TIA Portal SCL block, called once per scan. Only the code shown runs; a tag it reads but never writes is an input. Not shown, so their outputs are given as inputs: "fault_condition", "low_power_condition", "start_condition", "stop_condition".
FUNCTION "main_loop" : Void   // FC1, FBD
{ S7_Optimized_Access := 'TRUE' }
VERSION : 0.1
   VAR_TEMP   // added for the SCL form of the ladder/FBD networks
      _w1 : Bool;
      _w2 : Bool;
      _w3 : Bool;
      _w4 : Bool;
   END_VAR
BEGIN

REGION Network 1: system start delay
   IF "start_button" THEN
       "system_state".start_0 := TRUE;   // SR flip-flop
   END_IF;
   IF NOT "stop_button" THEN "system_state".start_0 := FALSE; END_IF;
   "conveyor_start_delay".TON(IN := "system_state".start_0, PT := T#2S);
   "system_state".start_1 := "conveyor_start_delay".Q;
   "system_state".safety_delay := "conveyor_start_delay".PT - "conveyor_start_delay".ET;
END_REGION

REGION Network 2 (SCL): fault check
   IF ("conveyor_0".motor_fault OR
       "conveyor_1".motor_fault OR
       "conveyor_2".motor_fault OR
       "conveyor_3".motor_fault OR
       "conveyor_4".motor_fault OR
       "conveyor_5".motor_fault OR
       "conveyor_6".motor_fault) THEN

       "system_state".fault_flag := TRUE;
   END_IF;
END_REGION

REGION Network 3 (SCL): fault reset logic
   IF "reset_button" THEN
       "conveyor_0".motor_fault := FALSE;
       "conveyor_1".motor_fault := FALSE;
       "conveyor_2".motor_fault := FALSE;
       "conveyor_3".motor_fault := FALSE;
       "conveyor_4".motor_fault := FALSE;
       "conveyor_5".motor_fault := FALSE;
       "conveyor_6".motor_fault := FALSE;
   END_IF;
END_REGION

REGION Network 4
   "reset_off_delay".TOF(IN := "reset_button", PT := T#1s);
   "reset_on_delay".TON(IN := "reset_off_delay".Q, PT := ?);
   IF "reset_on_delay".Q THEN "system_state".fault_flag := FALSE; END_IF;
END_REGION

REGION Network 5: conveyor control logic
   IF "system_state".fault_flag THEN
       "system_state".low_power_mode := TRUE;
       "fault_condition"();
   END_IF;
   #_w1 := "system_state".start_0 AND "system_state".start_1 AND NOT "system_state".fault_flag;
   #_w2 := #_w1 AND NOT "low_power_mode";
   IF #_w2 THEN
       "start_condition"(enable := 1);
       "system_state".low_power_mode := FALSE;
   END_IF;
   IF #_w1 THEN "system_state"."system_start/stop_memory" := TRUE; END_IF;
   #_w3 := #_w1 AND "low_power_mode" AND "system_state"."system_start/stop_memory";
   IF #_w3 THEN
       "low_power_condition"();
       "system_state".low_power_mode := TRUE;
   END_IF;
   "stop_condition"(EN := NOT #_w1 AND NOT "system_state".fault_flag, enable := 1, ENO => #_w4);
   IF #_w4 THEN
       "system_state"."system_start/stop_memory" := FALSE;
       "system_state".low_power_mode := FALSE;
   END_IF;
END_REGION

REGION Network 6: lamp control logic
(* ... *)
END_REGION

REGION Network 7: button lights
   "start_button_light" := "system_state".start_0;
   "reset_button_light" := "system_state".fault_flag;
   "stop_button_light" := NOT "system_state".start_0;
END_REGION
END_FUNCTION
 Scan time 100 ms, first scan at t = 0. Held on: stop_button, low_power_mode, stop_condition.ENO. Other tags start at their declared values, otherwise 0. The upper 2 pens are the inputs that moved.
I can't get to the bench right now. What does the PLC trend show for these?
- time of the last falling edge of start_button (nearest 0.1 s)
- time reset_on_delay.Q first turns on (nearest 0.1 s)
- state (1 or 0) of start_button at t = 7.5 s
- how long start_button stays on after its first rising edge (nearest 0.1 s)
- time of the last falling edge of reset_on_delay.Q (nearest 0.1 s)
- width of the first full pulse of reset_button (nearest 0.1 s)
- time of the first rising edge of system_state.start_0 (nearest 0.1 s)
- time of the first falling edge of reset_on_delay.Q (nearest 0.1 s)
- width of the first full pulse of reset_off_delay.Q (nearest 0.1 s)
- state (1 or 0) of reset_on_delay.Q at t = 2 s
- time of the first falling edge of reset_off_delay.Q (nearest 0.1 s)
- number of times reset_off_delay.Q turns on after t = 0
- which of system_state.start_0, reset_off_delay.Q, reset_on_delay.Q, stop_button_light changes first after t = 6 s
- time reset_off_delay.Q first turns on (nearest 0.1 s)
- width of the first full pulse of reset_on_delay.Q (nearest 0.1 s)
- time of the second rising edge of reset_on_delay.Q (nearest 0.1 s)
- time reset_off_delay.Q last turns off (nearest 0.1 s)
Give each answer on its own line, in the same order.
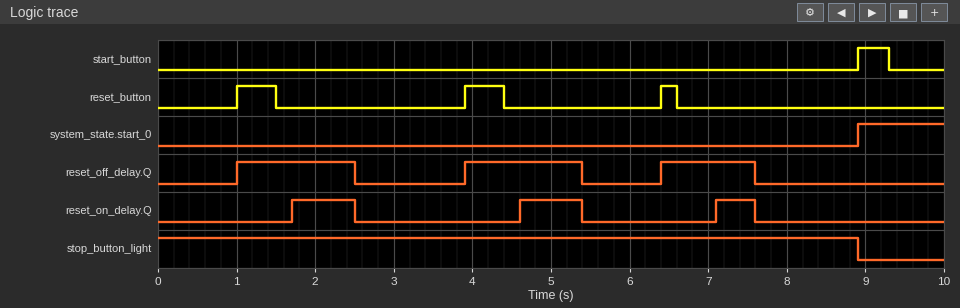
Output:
9.3 s
1.7 s
0
0.4 s
7.6 s
0.5 s
8.9 s
2.5 s
1.5 s
1
2.5 s
3
reset_off_delay.Q
1.0 s
0.8 s
4.6 s
7.6 s
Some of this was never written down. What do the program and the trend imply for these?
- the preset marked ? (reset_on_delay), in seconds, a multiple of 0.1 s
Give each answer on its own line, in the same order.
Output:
0.7 s
